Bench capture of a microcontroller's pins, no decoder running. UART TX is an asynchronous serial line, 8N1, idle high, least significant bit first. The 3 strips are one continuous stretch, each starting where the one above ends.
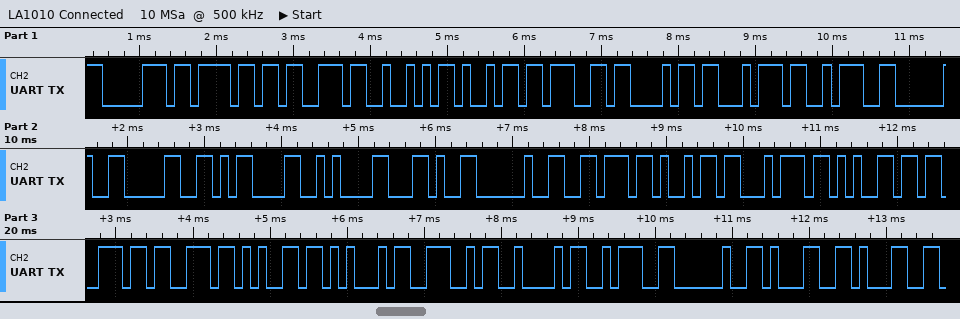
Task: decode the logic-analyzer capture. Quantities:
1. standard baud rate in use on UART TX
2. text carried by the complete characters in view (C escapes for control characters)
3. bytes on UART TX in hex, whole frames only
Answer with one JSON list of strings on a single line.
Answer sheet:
["9600 baud", "\"posRight: 0\\r\\n, vitesseENB: 11\"", "0x70 0x6F 0x73 0x52 0x69 0x67 0x68 0x74 0x3A 0x20 0x30 0x0D 0x0A 0x2C 0x20 0x76 0x69 0x74 0x65 0x73 0x73 0x65 0x45 0x4E 0x42 0x3A 0x20 0x31 0x31"]
